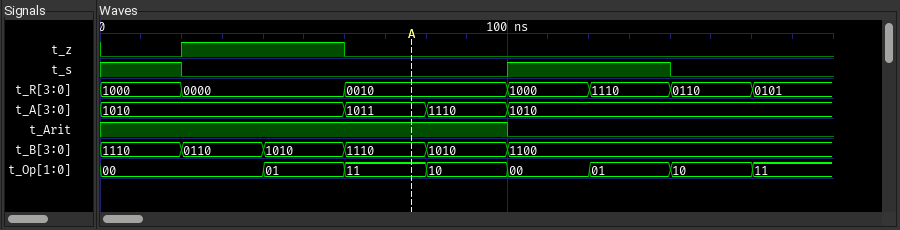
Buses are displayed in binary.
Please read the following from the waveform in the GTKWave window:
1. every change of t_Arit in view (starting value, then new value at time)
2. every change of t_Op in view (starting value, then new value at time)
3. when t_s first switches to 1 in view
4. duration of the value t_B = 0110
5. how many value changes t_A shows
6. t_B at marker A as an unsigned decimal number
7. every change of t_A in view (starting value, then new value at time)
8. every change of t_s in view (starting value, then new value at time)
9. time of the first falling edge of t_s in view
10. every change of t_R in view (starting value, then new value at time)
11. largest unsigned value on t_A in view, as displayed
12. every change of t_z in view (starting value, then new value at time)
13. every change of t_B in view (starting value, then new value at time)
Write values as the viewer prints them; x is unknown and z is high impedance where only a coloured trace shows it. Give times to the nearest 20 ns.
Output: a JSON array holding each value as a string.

["1, 0 at 100 ns", "00, 01 at 40 ns, 11 at 60 ns, 10 at 80 ns, 00 at 100 ns, 01 at 120 ns, 10 at 140 ns, 11 at 160 ns", "100 ns", "20 ns", "3", "14", "1010, 1011 at 60 ns, 1110 at 80 ns, 1010 at 100 ns", "1, 0 at 20 ns, 1 at 100 ns, 0 at 140 ns", "20 ns", "1000, 0000 at 20 ns, 0010 at 60 ns, 1000 at 100 ns, 1110 at 120 ns, 0110 at 140 ns, 0101 at 160 ns", "1110", "0, 1 at 20 ns, 0 at 60 ns", "1110, 0110 at 20 ns, 1010 at 40 ns, 1110 at 60 ns, 1010 at 80 ns, 1100 at 100 ns"]
